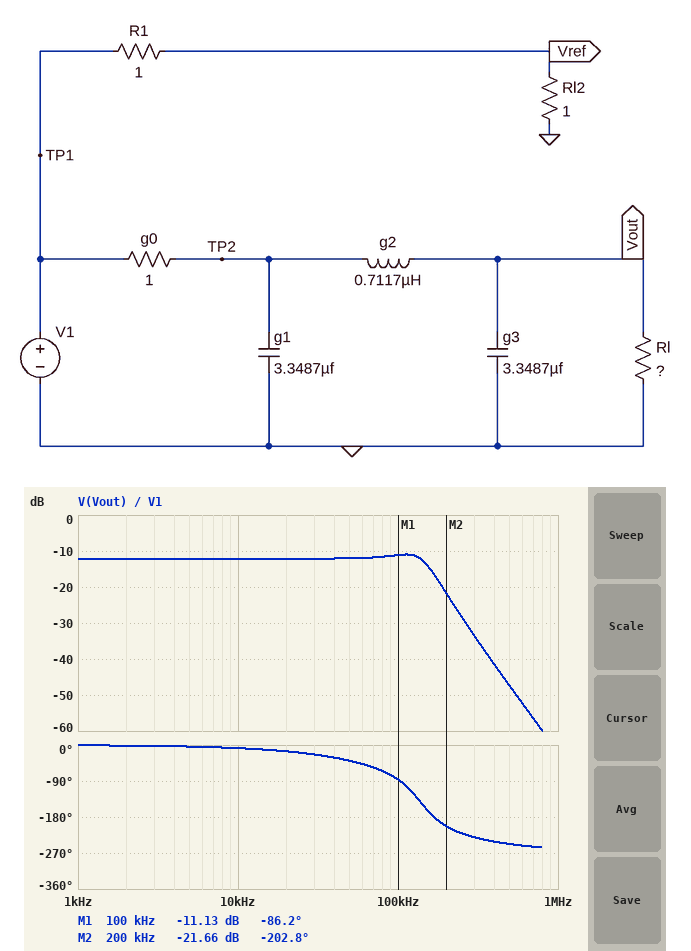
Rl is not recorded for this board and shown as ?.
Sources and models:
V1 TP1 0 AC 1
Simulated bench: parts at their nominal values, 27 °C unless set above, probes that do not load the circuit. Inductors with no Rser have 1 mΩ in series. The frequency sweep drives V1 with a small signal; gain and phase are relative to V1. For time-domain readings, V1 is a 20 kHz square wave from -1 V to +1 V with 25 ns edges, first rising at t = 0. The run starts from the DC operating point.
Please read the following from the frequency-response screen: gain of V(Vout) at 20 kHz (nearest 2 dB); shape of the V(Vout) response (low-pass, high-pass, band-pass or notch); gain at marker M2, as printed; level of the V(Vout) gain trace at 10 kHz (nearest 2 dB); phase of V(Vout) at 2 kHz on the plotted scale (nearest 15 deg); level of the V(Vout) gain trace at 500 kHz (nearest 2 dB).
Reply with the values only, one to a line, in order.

-12 dB
low-pass
-21.66 dB
-12 dB
0 deg
-48 dB
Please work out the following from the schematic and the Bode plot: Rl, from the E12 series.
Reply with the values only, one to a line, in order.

0.33 Ω
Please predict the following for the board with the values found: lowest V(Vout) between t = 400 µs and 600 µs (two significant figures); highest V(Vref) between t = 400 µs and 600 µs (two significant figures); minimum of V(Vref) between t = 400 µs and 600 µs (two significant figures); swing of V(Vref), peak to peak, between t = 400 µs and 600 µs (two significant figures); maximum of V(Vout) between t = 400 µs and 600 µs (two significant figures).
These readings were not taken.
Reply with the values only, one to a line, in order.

-330 mV
500 mV
-500 mV
1.0 V
330 mV
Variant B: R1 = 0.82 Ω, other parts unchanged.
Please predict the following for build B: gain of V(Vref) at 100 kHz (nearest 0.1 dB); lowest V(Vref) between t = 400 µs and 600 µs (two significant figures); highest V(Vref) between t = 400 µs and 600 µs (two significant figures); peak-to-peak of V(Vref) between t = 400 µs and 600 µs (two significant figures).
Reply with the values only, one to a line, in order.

-5.2 dB
-550 mV
550 mV
1.1 V
